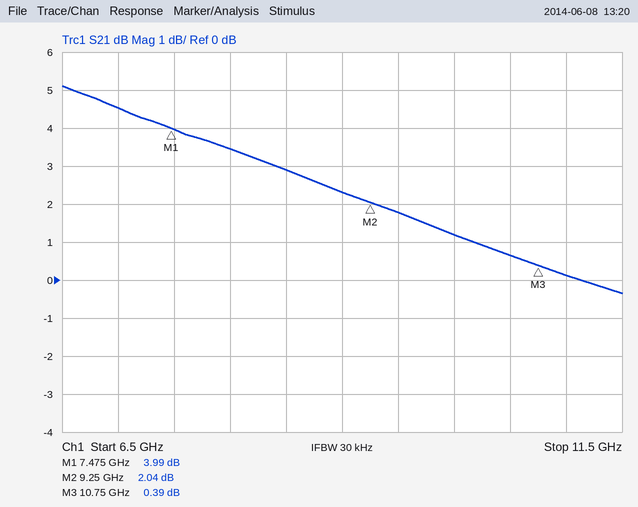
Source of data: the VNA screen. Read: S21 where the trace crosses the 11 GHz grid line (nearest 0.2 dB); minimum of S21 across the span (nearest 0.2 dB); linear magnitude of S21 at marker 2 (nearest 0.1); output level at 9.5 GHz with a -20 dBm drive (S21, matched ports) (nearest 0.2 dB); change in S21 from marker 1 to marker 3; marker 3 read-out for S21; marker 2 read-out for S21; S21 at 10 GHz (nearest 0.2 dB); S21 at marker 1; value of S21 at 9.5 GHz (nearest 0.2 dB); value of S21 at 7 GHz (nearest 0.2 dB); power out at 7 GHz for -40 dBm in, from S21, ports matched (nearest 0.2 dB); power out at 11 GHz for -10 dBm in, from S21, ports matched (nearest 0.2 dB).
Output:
0.2 dB
-0.4 dB
1.3
-18.2 dBm
-3.60 dB
0.39 dB
2.04 dB
1.2 dB
3.99 dB
1.8 dB
4.6 dB
-35.4 dBm
-9.8 dBm
